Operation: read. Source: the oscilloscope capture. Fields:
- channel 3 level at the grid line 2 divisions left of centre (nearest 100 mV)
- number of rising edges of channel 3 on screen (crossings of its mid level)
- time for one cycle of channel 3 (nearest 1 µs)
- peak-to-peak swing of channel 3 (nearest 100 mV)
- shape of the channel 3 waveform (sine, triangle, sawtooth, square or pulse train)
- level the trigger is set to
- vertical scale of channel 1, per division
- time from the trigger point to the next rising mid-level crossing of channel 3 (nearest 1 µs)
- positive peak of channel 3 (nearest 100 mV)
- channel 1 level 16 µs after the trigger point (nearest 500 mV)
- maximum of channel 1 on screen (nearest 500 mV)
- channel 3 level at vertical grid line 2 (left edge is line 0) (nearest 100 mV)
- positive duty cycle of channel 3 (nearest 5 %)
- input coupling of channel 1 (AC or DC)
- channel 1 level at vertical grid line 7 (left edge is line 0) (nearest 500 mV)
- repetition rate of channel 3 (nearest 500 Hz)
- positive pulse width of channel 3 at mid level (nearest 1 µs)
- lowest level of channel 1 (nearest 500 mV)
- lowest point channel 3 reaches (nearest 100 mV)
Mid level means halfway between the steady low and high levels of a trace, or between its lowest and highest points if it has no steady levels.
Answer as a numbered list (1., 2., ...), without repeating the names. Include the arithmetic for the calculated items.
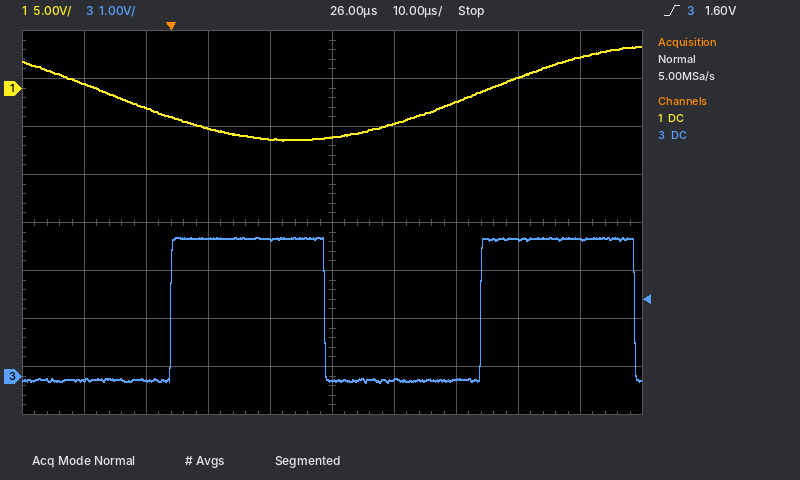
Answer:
1. 2.9 V
2. 2
3. 50 µs
4. 2.9 V − (-100 mV) = 3.0 V
5. square
6. 1.60 V
7. 5 V
8. 50 µs
9. 2.9 V
10. -5.5 V
11. 4.5 V
12. -100 mV
13. 25 µs / 50 µs ≈ 50 %
14. DC
15. -1.5 V
16. 1 / 50 µs ≈ 20.0 kHz
17. 25 µs
18. -5.5 V
19. -100 mV
